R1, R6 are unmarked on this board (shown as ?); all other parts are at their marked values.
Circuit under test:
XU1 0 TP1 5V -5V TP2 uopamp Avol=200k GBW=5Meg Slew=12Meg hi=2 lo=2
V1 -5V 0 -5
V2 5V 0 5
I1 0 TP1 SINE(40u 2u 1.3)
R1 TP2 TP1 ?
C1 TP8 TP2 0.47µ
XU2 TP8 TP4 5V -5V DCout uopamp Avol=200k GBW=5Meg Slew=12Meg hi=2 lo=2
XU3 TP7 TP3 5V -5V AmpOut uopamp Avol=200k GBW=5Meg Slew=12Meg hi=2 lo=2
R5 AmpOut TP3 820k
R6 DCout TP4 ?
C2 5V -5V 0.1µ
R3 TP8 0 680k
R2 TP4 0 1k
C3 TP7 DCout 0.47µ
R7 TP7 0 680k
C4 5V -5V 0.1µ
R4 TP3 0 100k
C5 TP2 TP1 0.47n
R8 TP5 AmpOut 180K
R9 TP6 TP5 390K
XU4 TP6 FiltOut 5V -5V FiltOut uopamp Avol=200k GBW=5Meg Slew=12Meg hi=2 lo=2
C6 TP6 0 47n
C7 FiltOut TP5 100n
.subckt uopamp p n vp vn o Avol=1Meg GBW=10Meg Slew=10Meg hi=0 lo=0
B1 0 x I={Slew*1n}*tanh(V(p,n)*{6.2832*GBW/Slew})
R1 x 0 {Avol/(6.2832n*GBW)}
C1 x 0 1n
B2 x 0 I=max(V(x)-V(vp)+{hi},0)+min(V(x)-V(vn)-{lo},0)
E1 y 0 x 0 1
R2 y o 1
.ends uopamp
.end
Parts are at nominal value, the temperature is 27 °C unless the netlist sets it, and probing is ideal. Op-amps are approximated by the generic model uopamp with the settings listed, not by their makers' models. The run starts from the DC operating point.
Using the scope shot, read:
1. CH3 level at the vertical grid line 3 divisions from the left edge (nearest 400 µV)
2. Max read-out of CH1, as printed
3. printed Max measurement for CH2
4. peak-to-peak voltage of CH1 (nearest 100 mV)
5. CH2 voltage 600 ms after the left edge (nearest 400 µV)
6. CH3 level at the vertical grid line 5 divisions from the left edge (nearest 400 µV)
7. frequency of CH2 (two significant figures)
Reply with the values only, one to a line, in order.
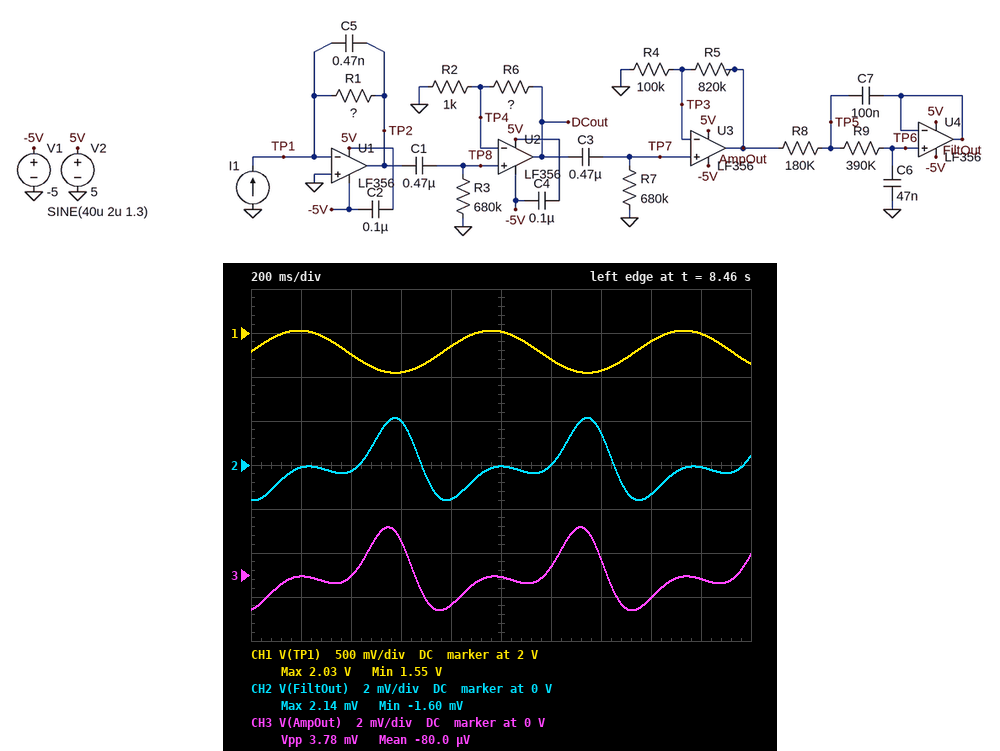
1.6 mV
2.03 V
2.14 mV
500 mV
2.0 mV
0 V
1.3 Hz
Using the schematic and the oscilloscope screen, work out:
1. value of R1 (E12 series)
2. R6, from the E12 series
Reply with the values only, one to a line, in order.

120 kΩ
120 kΩ
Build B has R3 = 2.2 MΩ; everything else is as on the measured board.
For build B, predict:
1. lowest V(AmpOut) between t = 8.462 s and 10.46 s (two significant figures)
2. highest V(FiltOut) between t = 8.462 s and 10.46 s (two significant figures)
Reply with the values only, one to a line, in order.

-1.5 mV
2.3 mV
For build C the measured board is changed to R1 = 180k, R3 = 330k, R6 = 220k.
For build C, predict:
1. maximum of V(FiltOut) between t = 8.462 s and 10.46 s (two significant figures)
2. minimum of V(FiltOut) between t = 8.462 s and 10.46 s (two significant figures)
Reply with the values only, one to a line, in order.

3.0 mV
-3.0 mV
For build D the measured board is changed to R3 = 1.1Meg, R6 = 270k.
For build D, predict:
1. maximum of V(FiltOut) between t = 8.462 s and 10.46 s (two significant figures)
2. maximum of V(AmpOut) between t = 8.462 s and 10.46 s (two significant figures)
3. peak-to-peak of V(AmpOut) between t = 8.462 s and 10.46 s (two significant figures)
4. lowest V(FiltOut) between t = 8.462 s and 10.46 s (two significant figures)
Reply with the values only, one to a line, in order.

5.0 mV
5.1 mV
8.5 mV
-3.4 mV
